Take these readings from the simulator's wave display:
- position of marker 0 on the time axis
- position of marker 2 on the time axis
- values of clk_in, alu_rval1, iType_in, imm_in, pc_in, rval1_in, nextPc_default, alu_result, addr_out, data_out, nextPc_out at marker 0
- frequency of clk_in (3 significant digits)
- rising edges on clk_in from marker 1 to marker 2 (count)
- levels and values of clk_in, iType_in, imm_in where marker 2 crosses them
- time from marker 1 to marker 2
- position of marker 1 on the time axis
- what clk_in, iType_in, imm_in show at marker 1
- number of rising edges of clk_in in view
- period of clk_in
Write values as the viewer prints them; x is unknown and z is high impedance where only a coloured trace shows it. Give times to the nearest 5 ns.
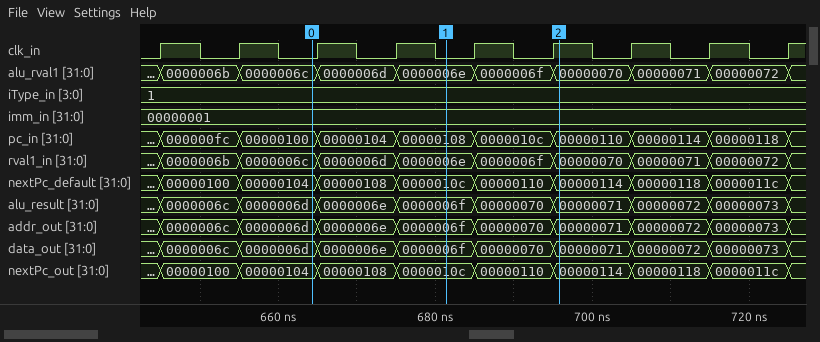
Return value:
665 ns
695 ns
clk_in=0, alu_rval1=0000006c, iType_in=1, imm_in=00000001, pc_in=00000100, rval1_in=0000006c, nextPc_default=00000104, alu_result=0000006d, addr_out=0000006d, data_out=0000006d, nextPc_out=00000104
100 MHz
2
clk_in=1, iType_in=1, imm_in=00000001
15 ns
680 ns
clk_in=0, iType_in=1, imm_in=00000001
9
10 ns
